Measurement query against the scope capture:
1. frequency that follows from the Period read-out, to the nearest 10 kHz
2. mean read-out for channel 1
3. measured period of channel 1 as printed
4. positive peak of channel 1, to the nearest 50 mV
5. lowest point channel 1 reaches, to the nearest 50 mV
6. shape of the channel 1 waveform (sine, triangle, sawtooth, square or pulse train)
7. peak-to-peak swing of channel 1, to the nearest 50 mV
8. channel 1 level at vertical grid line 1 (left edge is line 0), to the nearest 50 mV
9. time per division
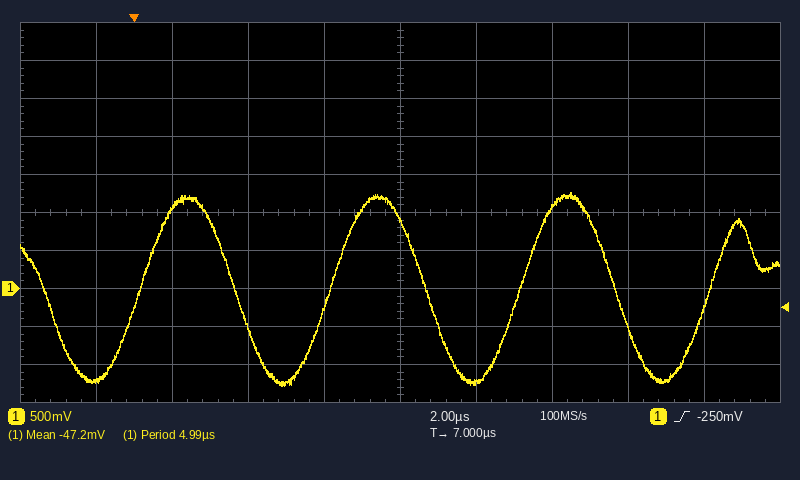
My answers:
200 kHz
-47.2 mV
4.99 µs
1.25 V
-1.30 V
sine
2.55 V
-1.20 V
2 µs
